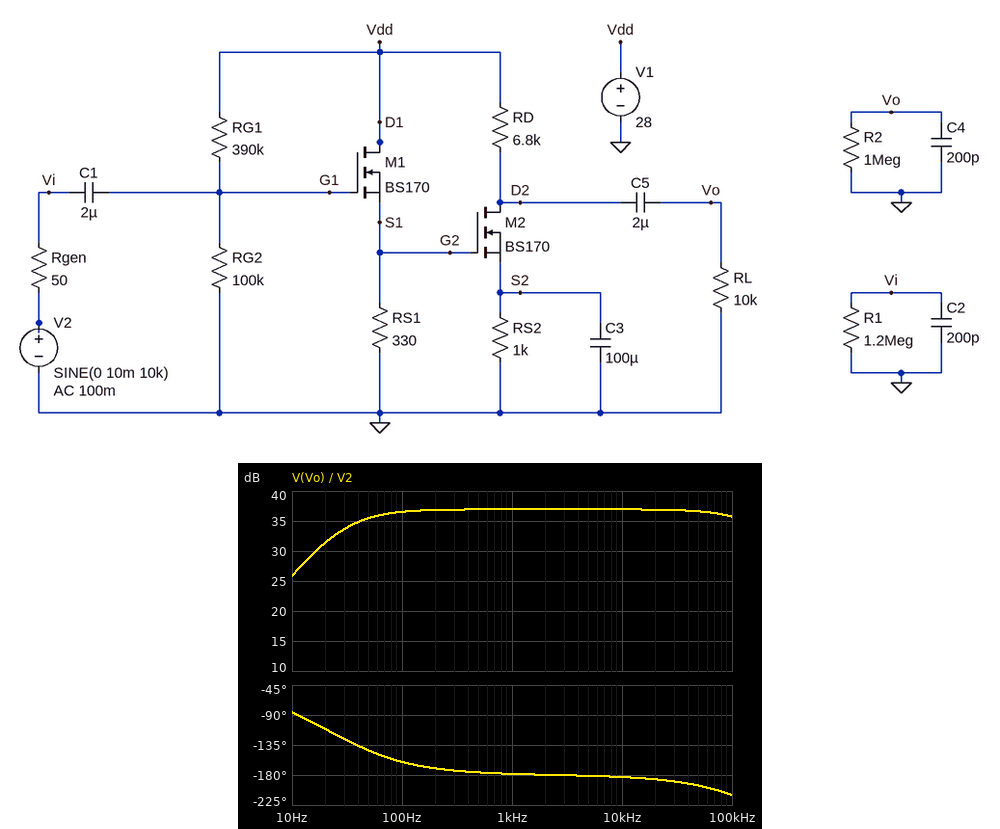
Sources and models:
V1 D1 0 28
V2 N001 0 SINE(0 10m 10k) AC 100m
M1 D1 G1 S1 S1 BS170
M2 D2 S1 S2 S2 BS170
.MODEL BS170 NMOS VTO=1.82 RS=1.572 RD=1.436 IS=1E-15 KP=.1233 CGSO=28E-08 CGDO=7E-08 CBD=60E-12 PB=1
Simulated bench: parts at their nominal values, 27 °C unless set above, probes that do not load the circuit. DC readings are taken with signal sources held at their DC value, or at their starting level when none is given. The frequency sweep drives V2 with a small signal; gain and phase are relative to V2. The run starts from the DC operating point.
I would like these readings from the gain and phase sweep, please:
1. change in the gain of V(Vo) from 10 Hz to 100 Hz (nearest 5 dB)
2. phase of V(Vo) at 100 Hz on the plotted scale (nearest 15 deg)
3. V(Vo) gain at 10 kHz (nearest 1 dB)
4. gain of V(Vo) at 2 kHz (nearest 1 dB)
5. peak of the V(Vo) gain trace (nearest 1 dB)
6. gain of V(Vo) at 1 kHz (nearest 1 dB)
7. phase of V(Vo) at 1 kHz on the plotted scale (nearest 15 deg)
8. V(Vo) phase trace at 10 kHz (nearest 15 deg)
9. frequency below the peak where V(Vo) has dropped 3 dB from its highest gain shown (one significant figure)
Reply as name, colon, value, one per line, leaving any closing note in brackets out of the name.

change in the gain of V(Vo) from 10 Hz to 100 Hz: 10 dB
phase of V(Vo) at 100 Hz on the plotted scale: -165 deg
V(Vo) gain at 10 kHz: 37 dB
gain of V(Vo) at 2 kHz: 37 dB
peak of the V(Vo) gain trace: 37 dB
gain of V(Vo) at 1 kHz: 37 dB
phase of V(Vo) at 1 kHz on the plotted scale: -180 deg
V(Vo) phase trace at 10 kHz: -180 deg
frequency below the peak where V(Vo) has dropped 3 dB from its highest gain shown: 30 Hz
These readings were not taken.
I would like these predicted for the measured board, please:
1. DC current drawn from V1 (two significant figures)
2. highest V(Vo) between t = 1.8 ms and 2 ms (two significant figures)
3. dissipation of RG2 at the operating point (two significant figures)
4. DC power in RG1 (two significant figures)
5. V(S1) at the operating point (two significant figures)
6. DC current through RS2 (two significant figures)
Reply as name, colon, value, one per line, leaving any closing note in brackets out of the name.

DC current drawn from V1: 12 mA
highest V(Vo) between t = 1.8 ms and 2 ms: 690 mV
dissipation of RG2 at the operating point: 330 µW
DC power in RG1: 1.3 mW
V(S1) at the operating point: 3.5 V
DC current through RS2: 1.5 mA
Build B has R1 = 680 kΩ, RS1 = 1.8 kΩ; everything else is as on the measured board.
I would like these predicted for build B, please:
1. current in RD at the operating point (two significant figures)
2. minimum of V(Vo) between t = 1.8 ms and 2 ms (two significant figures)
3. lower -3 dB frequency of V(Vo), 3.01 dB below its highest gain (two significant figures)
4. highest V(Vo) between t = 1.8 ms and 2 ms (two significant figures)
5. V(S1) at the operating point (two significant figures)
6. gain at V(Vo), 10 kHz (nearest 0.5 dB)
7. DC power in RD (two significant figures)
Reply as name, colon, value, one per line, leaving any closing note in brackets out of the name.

current in RD at the operating point: 1.7 mA
minimum of V(Vo) between t = 1.8 ms and 2 ms: -800 mV
lower -3 dB frequency of V(Vo), 3.01 dB below its highest gain: 34 Hz
highest V(Vo) between t = 1.8 ms and 2 ms: 770 mV
V(S1) at the operating point: 3.7 V
gain at V(Vo), 10 kHz: 38.0 dB
DC power in RD: 20 mW
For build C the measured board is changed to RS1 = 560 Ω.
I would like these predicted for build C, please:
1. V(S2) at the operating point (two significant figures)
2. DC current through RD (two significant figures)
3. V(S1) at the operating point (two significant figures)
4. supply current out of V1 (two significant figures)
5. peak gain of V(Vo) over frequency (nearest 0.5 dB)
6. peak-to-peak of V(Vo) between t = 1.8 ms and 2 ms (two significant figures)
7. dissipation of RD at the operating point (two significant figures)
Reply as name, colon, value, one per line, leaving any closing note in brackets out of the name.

V(S2) at the operating point: 1.6 V
DC current through RD: 1.6 mA
V(S1) at the operating point: 3.6 V
supply current out of V1: 8.0 mA
peak gain of V(Vo) over frequency: 37.5 dB
peak-to-peak of V(Vo) between t = 1.8 ms and 2 ms: 1.5 V
dissipation of RD at the operating point: 17 mW
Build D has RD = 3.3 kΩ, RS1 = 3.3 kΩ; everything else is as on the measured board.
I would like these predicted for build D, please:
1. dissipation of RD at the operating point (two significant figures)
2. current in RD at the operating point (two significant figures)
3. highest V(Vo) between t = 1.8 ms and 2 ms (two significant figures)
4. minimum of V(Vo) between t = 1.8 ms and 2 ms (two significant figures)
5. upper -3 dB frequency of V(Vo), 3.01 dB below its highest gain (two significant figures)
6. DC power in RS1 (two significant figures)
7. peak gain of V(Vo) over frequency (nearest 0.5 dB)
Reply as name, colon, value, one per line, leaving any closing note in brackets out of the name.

dissipation of RD at the operating point: 10 mW
current in RD at the operating point: 1.8 mA
highest V(Vo) between t = 1.8 ms and 2 ms: 480 mV
minimum of V(Vo) between t = 1.8 ms and 2 ms: -500 mV
upper -3 dB frequency of V(Vo), 3.01 dB below its highest gain: 280 kHz
DC power in RS1: 4.3 mW
peak gain of V(Vo) over frequency: 34.0 dB
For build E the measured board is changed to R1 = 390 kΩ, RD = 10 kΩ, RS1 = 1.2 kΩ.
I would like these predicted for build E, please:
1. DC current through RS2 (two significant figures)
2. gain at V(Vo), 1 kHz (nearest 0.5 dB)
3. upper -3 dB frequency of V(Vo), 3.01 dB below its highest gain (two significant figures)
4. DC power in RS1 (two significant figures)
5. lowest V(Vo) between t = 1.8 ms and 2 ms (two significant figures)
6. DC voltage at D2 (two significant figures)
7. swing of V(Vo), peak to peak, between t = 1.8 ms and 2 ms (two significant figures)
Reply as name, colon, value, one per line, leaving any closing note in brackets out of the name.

DC current through RS2: 1.7 mA
gain at V(Vo), 1 kHz: 39.5 dB
upper -3 dB frequency of V(Vo), 3.01 dB below its highest gain: 140 kHz
DC power in RS1: 11 mW
lowest V(Vo) between t = 1.8 ms and 2 ms: -970 mV
DC voltage at D2: 11 V
swing of V(Vo), peak to peak, between t = 1.8 ms and 2 ms: 1.9 V
